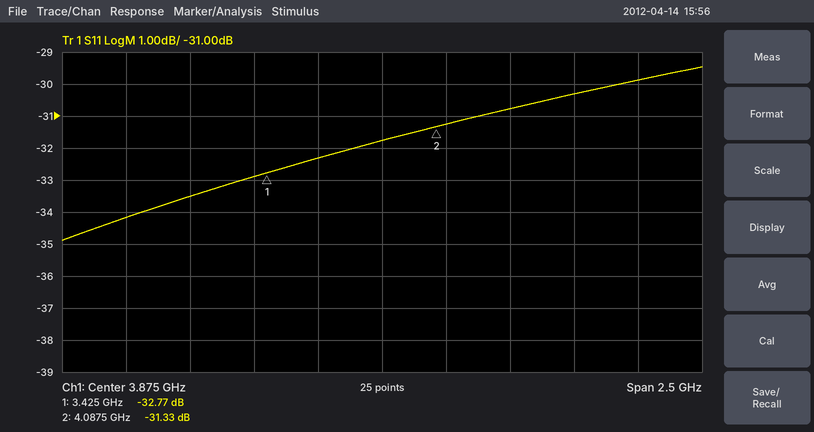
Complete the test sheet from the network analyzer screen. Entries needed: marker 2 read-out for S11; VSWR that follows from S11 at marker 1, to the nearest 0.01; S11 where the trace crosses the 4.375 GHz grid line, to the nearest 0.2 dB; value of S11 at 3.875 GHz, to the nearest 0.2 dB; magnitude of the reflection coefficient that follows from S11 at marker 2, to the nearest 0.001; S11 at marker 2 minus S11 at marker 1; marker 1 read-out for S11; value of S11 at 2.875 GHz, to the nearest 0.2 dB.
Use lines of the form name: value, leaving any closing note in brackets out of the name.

marker 2 read-out for S11: -31.33 dB
VSWR that follows from S11 at marker 1, to the nearest 0.01: 1.05
S11 where the trace crosses the 4.375 GHz grid line, to the nearest 0.2 dB: -30.8 dB
value of S11 at 3.875 GHz, to the nearest 0.2 dB: -31.8 dB
magnitude of the reflection coefficient that follows from S11 at marker 2, to the nearest 0.001: 0.027
S11 at marker 2 minus S11 at marker 1: 1.44 dB
marker 1 read-out for S11: -32.77 dB
value of S11 at 2.875 GHz, to the nearest 0.2 dB: -34.2 dB
